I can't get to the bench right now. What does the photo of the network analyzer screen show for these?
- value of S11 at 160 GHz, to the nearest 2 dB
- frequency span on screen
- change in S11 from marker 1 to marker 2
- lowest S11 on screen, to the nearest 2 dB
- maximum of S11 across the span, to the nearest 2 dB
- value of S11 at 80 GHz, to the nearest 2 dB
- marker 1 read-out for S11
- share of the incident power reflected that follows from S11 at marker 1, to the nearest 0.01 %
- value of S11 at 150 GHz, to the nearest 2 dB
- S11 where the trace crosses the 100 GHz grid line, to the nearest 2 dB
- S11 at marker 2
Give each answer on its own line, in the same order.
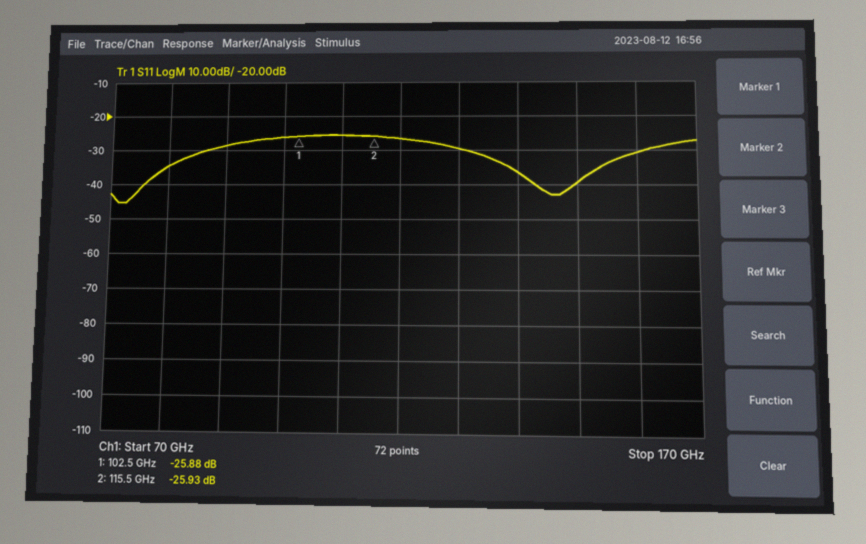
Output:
-30 dB
100 GHz
-0.05 dB
-46 dB
-26 dB
-34 dB
-25.88 dB
0.26 %
-40 dB
-26 dB
-25.93 dB
